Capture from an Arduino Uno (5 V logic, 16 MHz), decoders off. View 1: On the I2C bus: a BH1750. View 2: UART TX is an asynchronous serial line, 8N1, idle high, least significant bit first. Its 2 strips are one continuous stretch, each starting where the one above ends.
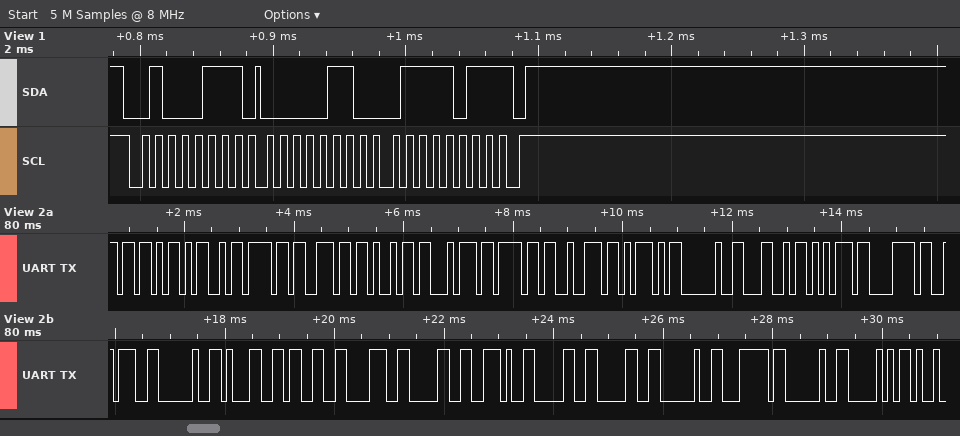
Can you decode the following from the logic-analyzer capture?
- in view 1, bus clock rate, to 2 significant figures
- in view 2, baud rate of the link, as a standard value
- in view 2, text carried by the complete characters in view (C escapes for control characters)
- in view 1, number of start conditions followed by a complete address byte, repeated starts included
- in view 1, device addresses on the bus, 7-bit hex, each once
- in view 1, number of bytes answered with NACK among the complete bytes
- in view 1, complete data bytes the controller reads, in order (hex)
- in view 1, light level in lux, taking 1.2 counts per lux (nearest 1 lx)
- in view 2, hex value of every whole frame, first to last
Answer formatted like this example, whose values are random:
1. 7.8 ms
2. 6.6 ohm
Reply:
1. 100 kHz
2. 9600 baud
3. "[Monitor] Lux: 1380.00 | P"
4. 1
5. 0x23
6. 1
7. 06 7B
8. 1382 lx
9. 5B 4D 6F 6E 69 74 6F 72 5D 20 4C 75 78 3A 20 31 33 38 30 2E 30 30 20 7C 20 50
